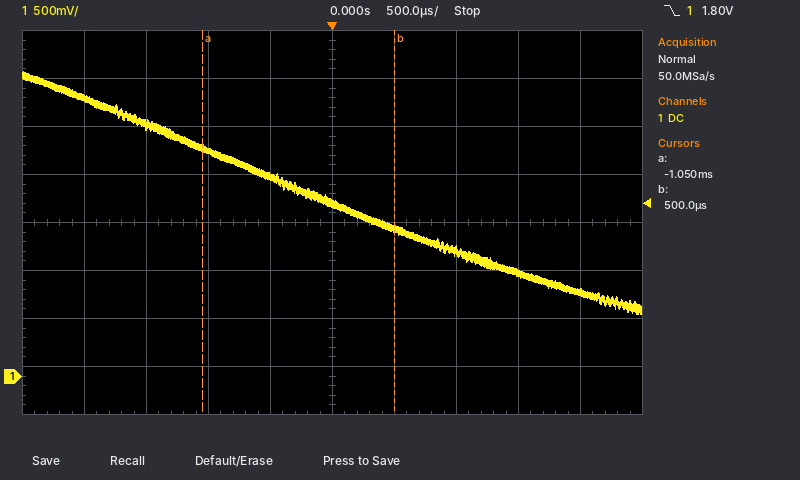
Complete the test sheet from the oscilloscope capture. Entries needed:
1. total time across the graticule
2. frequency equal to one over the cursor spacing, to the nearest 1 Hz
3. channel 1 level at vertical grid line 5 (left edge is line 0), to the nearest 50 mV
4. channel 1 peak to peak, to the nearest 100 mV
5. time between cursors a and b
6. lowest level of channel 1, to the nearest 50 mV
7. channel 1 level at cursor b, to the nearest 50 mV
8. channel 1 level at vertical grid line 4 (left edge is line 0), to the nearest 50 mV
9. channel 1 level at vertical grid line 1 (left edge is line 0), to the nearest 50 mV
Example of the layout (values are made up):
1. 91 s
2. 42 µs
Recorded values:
1. 5 ms
2. 645 Hz
3. 1.80 V
4. 2.50 V
5. 1.55 ms
6. 650 mV
7. 1.55 V
8. 2.10 V
9. 2.90 V
